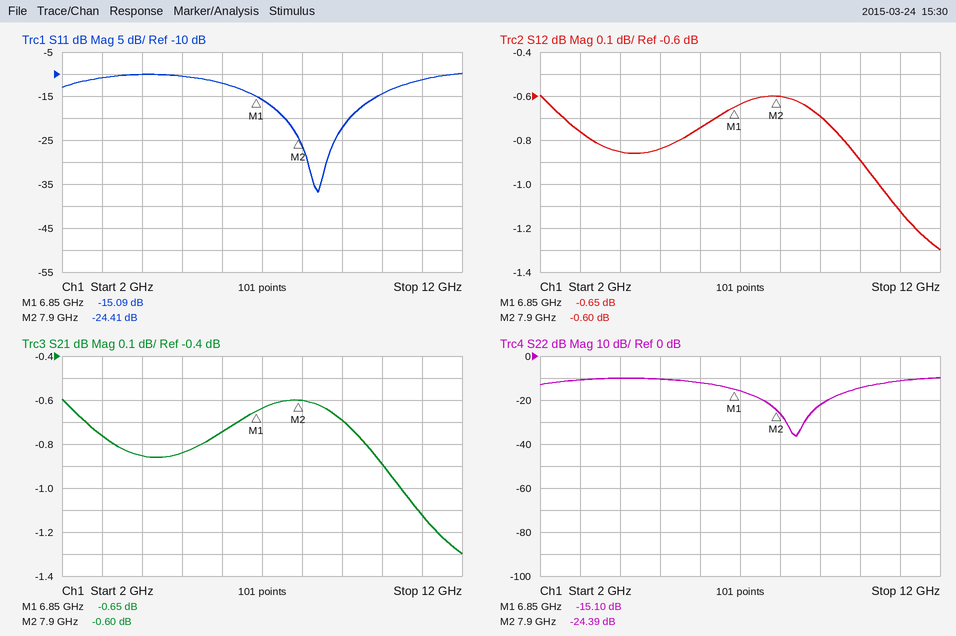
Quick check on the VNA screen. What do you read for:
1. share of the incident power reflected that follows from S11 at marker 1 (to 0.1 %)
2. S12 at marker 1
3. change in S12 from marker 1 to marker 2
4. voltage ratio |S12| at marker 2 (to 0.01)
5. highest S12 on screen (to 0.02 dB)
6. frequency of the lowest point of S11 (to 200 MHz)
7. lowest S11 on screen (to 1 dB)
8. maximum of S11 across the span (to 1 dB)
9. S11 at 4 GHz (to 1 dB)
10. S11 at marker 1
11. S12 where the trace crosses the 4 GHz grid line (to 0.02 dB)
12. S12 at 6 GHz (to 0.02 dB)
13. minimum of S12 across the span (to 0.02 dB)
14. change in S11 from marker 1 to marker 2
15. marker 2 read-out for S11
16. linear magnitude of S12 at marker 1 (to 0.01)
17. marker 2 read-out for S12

3.1 %
-0.65 dB
0.05 dB
0.93
-0.60 dB
8.4 GHz
-37 dB
-10 dB
-10 dB
-15.09 dB
-0.86 dB
-0.74 dB
-1.30 dB
-9.32 dB
-24.41 dB
0.93
-0.60 dB
